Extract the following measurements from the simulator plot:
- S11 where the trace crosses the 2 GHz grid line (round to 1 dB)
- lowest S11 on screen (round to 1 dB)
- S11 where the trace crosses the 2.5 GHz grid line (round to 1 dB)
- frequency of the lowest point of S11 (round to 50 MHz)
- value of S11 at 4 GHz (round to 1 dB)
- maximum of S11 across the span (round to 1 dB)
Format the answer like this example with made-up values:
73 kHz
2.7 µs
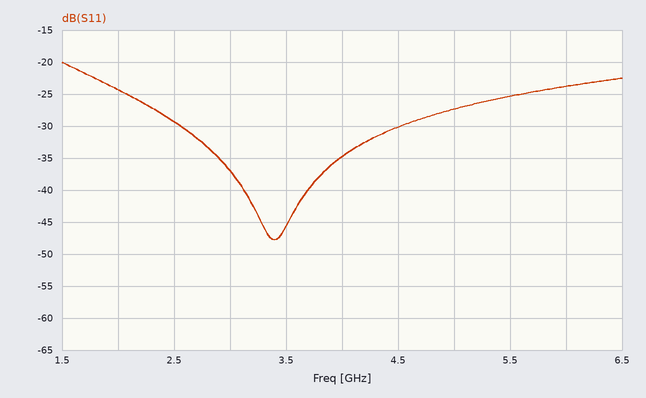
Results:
-24 dB
-48 dB
-29 dB
3.40 GHz
-35 dB
-20 dB
